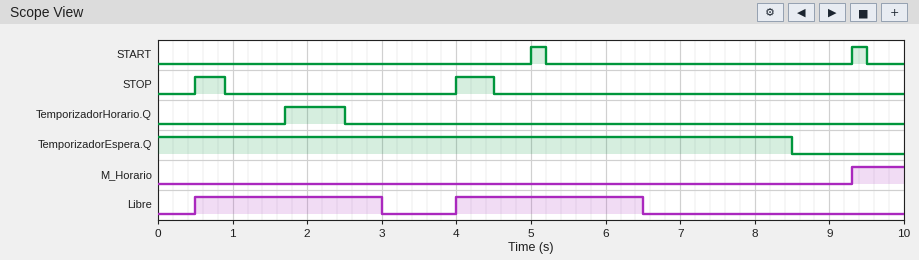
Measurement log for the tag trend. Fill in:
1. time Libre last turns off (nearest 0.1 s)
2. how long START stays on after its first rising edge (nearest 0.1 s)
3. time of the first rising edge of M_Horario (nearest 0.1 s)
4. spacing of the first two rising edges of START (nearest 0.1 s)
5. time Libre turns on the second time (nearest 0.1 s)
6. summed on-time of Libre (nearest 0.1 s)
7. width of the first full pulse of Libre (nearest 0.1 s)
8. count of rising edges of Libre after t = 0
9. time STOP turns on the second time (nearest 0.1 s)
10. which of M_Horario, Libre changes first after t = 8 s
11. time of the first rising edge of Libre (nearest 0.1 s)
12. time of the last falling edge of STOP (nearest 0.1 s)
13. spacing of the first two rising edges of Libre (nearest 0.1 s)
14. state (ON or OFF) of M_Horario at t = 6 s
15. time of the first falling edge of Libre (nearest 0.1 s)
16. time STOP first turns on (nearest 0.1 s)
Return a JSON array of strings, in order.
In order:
["6.5 s", "0.2 s", "9.3 s", "4.3 s", "4.0 s", "5.0 s", "2.5 s", "2", "4.0 s", "M_Horario", "0.5 s", "4.5 s", "3.5 s", "OFF", "3.0 s", "0.5 s"]
